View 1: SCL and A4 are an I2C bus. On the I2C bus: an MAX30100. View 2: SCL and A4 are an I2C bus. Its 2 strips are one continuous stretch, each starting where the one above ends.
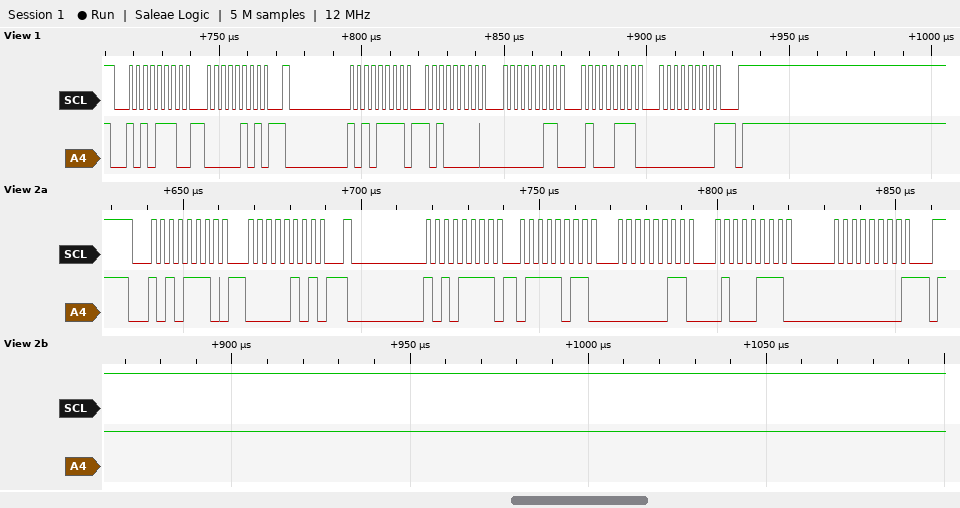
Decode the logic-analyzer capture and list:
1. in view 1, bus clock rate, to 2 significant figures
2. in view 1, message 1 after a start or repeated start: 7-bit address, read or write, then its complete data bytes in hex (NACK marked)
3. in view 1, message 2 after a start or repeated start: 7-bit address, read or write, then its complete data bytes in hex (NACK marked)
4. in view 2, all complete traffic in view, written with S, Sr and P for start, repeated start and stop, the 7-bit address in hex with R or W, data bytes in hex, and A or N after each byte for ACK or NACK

400 kHz
0x57 write: 05
0x57 read: A0 03 47 00 NACK
S 57W A 05 A Sr 57R A 7B A 03 A 47 A 00 N P
